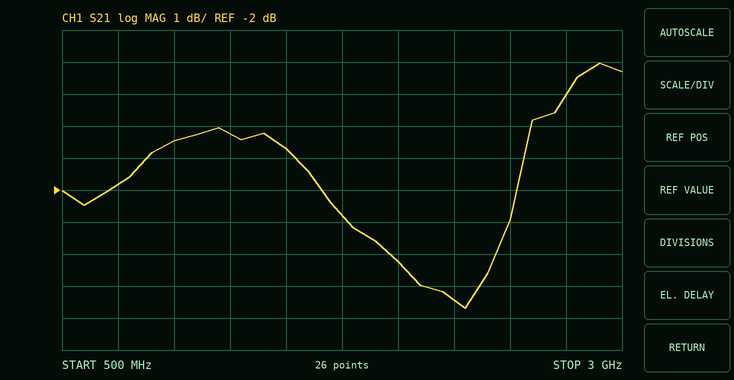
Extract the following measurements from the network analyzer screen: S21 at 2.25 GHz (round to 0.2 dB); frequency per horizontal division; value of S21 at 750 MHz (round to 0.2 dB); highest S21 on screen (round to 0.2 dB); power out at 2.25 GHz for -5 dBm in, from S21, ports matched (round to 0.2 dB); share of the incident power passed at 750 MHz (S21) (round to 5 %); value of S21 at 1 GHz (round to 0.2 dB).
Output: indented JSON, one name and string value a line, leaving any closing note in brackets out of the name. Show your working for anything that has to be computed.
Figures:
{
  "S21 at 2.25 GHz": "-5.4 dB",
  "frequency per horizontal division": "250 MHz",
  "value of S21 at 750 MHz": "-1.8 dB",
  "highest S21 on screen": "2.0 dB",
  "power out at 2.25 GHz for -5 dBm in, from S21, ports matched": "-5 dBm + (-5.4 dB) = -10.4 dBm",
  "share of the incident power passed at 750 MHz (S21)": "10^(-1.8/10) ≈ 66.1 %, so 65 % to the nearest 5 %",
  "value of S21 at 1 GHz": "-0.4 dB"
}
